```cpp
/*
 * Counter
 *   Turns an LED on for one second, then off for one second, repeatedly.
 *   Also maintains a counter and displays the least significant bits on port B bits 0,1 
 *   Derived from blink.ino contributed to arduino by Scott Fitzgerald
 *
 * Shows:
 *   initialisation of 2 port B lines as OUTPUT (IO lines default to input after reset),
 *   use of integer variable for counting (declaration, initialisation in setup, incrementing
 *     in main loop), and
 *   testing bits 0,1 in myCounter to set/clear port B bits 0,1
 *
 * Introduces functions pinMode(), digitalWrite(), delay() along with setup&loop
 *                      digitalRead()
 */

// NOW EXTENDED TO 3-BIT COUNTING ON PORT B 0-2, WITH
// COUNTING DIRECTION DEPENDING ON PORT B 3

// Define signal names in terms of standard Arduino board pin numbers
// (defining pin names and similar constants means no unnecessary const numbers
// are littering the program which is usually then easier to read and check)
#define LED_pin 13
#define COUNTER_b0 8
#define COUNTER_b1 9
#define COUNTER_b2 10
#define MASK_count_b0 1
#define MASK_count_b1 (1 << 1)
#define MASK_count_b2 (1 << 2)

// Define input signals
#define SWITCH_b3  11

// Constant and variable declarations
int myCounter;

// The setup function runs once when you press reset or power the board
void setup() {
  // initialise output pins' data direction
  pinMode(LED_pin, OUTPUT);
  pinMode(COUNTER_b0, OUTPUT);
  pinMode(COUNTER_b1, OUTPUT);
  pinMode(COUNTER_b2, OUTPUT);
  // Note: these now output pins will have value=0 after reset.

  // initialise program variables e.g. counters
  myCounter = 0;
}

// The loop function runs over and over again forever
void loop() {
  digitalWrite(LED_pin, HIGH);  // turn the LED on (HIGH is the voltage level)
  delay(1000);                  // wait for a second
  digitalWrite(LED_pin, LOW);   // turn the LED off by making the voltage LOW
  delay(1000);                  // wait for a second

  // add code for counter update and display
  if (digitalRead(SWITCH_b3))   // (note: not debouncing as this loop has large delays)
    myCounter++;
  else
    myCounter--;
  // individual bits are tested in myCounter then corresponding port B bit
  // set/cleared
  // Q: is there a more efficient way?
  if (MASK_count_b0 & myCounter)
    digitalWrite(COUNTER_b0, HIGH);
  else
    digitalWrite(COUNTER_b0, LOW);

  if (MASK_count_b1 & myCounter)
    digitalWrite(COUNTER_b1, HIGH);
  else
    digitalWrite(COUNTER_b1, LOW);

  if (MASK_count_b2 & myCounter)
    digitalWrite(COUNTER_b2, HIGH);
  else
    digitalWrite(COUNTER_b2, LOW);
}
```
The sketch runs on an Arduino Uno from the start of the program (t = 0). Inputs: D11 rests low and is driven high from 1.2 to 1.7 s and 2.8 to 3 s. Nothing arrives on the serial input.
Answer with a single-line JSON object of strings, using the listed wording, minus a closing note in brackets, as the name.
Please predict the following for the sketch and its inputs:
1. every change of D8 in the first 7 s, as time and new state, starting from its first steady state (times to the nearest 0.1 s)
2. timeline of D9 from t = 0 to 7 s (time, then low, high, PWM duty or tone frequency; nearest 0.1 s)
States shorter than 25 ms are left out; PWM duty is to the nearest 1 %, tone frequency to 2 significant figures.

{"every change of D8 in the first 7 s, as time and new state, starting from its first steady state": "0 s low; 2 s high; 4 s low; 6 s high", "timeline of D9 from t = 0 to 7 s": "0 s low; 2 s high; 6 s low"}
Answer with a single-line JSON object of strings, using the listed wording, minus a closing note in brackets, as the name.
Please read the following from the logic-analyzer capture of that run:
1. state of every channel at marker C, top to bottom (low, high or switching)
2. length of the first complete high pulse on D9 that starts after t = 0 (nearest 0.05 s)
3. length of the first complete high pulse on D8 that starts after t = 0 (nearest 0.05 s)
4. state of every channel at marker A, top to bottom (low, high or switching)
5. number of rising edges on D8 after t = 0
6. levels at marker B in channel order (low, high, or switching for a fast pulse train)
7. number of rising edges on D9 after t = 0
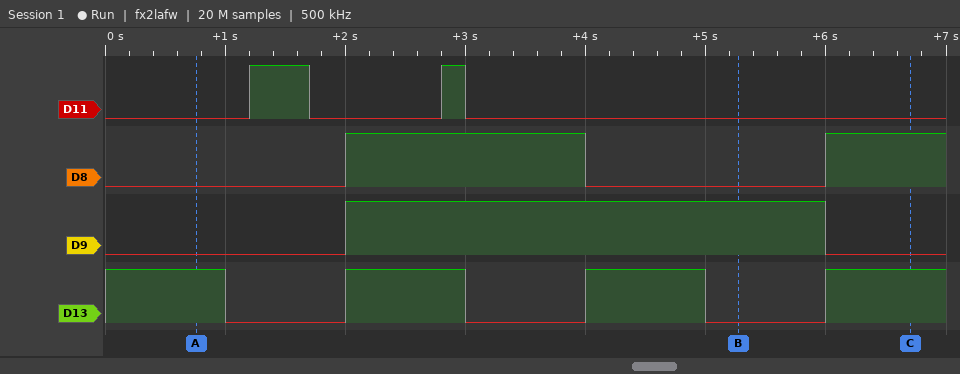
{"state of every channel at marker C, top to bottom": "D11 low, D8 high, D9 low, D13 high", "length of the first complete high pulse on D9 that starts after t = 0": "4.00 s", "length of the first complete high pulse on D8 that starts after t = 0": "2.00 s", "state of every channel at marker A, top to bottom": "D11 low, D8 low, D9 low, D13 high", "number of rising edges on D8 after t = 0": "2", "levels at marker B in channel order": "D11 low, D8 low, D9 high, D13 low", "number of rising edges on D9 after t = 0": "1"}
